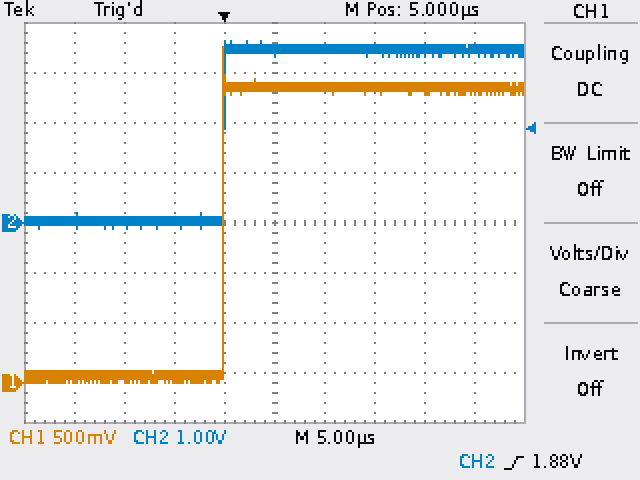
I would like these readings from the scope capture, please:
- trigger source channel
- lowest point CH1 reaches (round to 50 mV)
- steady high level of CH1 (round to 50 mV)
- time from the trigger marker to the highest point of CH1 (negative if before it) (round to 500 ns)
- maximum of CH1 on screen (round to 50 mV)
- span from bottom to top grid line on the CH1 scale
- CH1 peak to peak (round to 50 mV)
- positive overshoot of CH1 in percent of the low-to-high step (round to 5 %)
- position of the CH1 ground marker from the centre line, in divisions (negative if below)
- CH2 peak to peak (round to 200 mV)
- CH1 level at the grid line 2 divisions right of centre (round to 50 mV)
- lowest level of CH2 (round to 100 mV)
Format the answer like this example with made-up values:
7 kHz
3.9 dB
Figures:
CH2
0 mV
2.95 V
0.0 µs
3.35 V
4 V
3.35 V
15 %
-3.2 div
3.8 V
2.95 V
-100 mV
